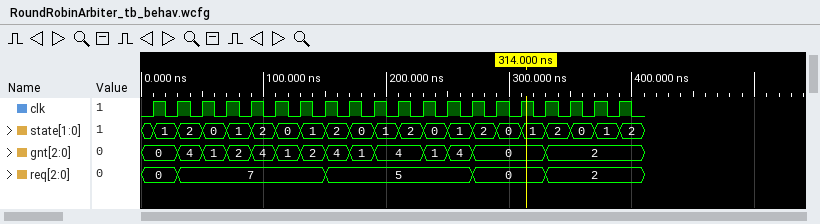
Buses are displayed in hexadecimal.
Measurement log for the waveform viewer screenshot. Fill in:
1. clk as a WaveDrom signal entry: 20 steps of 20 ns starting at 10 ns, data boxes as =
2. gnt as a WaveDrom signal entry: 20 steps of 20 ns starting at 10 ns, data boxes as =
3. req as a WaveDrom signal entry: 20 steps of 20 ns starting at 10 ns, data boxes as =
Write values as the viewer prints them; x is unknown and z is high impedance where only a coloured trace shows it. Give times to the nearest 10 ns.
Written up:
{name: 'clk', wave: 'p...................'}
{name: 'gnt', wave: '==========.===..=...', data: '0 4 1 2 4 1 2 4 1 4 1 4 0 2'}
{name: 'req', wave: '==.....=.....=..=...', data: '0 7 5 0 2'}
